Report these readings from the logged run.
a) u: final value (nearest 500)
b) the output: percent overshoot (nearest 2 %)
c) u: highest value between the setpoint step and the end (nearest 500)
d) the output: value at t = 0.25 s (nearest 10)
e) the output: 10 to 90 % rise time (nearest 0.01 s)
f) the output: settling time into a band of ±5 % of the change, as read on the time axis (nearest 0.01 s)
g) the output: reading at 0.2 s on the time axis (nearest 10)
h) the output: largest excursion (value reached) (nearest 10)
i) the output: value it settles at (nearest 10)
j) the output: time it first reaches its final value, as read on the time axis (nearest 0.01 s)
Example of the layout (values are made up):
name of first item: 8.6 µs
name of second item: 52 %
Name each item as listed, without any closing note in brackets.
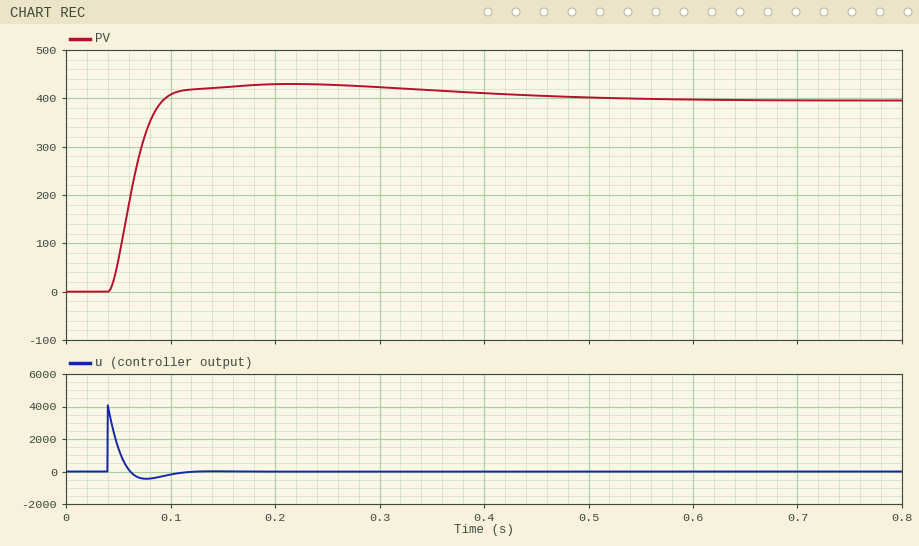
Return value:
u: final value: 0
the output: percent overshoot: 8 %
u: highest value between the setpoint step and the end: 4000
the output: value at t = 0.25 s: 430
the output: 10 to 90 % rise time: 0.03 s
the output: settling time into a band of ±5 % of the change, as read on the time axis: 0.36 s
the output: reading at 0.2 s on the time axis: 430
the output: largest excursion (value reached): 430
the output: value it settles at: 400
the output: time it first reaches its final value, as read on the time axis: 0.09 s
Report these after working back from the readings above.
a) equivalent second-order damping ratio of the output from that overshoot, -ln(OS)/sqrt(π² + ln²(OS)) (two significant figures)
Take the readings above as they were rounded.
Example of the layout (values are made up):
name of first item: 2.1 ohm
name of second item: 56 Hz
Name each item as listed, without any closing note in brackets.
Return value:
equivalent second-order damping ratio of the output from that overshoot, -ln(OS)/sqrt(π² + ln²(OS)): 0.63
